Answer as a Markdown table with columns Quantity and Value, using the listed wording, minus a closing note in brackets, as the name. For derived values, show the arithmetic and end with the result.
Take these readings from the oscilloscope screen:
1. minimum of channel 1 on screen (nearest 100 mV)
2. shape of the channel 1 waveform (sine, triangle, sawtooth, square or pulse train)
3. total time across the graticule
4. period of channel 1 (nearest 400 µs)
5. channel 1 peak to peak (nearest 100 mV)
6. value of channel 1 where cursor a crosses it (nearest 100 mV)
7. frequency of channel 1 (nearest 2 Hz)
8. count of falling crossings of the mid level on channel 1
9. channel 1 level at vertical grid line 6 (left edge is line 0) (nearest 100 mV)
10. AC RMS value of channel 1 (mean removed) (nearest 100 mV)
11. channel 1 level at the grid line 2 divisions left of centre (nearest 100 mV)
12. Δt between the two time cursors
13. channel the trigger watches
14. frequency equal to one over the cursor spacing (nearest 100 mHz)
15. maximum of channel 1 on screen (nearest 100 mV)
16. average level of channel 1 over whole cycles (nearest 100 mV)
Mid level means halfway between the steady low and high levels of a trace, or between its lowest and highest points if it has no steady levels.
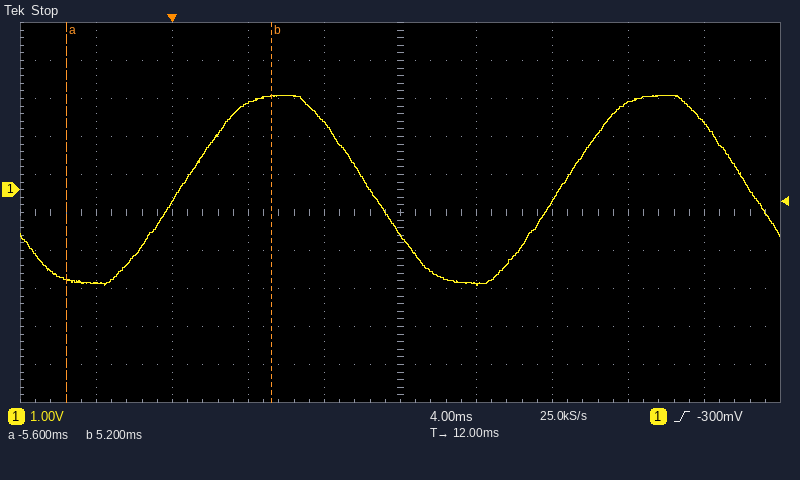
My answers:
| Quantity | Value |
|---|---|
| minimum of channel 1 on screen | -2.5 V |
| shape of the channel 1 waveform | sine |
| total time across the graticule | 40 ms |
| period of channel 1 | 20.0 ms |
| channel 1 peak to peak | 2.5 V − (-2.5 V) = 5.0 V |
| value of channel 1 where cursor a crosses it | -2.4 V |
| frequency of channel 1 | 1 / 20.0 ms ≈ 50 Hz |
| count of falling crossings of the mid level on channel 1 | 2 |
| channel 1 level at vertical grid line 6 (left edge is line 0) | -2.5 V |
| AC RMS value of channel 1 (mean removed) | 5.0 V / (2√2) ≈ 1.8 V |
| channel 1 level at the grid line 2 divisions left of centre | 2.3 V |
| Δt between the two time cursors | 5.2 ms − (-5.6 ms) = 10.8 ms |
| channel the trigger watches | channel 1 |
| frequency equal to one over the cursor spacing | 1 / 10.8 ms ≈ 92.6 Hz |
| maximum of channel 1 on screen | 2.5 V |
| average level of channel 1 over whole cycles | (2.5 V + (-2.5 V)) / 2 ≈ 0.0 V |
